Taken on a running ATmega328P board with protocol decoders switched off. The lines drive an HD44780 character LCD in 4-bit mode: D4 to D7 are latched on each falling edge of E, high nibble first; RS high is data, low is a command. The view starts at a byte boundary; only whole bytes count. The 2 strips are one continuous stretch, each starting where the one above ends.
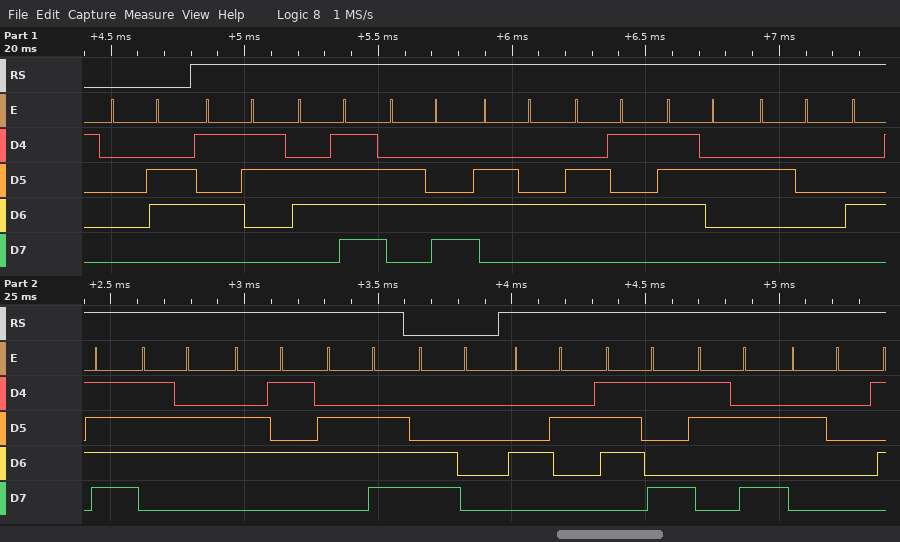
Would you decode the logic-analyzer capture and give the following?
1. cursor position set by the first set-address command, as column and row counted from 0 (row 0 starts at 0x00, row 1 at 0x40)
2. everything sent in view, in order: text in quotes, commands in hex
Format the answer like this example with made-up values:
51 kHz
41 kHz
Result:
column 0, row 1
0x06 "Solder Oven" 0xC0 "By: "
